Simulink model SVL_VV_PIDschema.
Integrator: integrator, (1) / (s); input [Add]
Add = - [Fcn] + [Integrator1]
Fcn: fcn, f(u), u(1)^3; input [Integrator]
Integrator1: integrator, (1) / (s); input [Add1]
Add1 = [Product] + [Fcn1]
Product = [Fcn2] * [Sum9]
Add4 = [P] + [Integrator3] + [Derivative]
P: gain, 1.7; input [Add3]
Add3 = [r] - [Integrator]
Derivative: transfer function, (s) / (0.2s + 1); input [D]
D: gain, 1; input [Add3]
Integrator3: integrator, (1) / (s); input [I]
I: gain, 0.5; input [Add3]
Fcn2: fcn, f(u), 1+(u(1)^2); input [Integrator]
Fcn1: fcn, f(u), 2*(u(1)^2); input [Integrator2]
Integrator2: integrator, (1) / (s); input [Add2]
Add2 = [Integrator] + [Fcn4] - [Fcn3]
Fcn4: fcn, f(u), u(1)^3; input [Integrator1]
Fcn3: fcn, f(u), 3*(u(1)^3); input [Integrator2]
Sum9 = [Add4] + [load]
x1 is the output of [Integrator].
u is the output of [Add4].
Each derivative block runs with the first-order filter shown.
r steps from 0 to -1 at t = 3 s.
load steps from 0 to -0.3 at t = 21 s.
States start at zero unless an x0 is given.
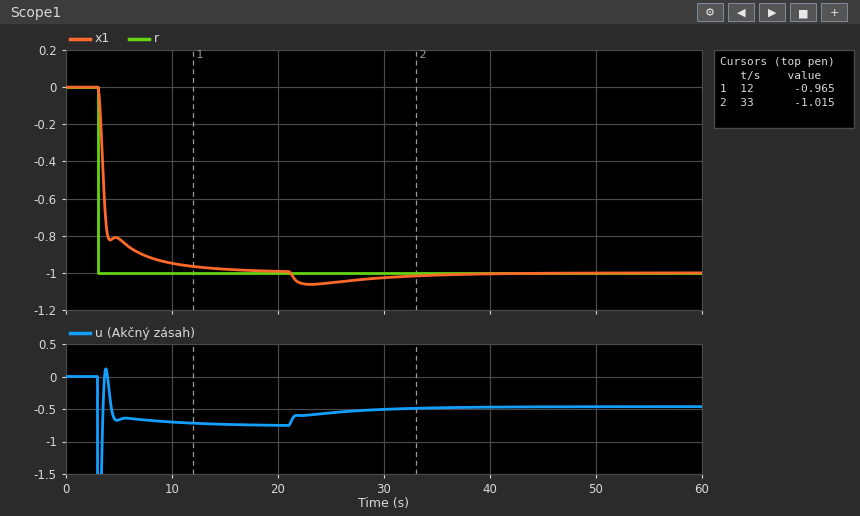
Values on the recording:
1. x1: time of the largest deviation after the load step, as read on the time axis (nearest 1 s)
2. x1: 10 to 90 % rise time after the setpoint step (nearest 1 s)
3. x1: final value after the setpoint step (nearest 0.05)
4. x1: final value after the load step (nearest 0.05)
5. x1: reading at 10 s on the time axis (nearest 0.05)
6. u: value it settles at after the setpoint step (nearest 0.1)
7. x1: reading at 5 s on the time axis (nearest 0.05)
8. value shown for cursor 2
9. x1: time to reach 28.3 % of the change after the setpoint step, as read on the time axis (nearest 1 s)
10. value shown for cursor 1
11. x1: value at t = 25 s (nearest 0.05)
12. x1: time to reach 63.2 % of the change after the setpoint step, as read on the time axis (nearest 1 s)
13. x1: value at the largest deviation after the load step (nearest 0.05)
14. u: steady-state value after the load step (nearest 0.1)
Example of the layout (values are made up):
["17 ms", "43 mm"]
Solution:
["23 s", "4 s", "-1.00", "-1.00", "-0.95", "-0.8", "-0.80", "-1.015", "3 s", "-0.965", "-1.05", "4 s", "-1.05", "-0.5"]
